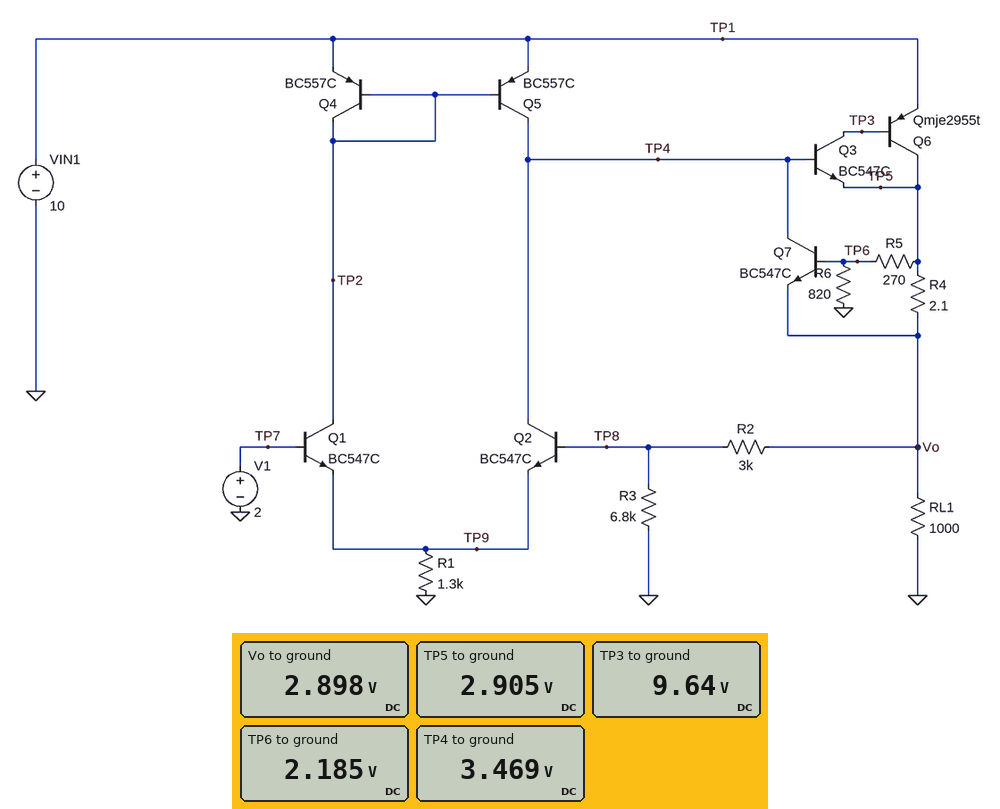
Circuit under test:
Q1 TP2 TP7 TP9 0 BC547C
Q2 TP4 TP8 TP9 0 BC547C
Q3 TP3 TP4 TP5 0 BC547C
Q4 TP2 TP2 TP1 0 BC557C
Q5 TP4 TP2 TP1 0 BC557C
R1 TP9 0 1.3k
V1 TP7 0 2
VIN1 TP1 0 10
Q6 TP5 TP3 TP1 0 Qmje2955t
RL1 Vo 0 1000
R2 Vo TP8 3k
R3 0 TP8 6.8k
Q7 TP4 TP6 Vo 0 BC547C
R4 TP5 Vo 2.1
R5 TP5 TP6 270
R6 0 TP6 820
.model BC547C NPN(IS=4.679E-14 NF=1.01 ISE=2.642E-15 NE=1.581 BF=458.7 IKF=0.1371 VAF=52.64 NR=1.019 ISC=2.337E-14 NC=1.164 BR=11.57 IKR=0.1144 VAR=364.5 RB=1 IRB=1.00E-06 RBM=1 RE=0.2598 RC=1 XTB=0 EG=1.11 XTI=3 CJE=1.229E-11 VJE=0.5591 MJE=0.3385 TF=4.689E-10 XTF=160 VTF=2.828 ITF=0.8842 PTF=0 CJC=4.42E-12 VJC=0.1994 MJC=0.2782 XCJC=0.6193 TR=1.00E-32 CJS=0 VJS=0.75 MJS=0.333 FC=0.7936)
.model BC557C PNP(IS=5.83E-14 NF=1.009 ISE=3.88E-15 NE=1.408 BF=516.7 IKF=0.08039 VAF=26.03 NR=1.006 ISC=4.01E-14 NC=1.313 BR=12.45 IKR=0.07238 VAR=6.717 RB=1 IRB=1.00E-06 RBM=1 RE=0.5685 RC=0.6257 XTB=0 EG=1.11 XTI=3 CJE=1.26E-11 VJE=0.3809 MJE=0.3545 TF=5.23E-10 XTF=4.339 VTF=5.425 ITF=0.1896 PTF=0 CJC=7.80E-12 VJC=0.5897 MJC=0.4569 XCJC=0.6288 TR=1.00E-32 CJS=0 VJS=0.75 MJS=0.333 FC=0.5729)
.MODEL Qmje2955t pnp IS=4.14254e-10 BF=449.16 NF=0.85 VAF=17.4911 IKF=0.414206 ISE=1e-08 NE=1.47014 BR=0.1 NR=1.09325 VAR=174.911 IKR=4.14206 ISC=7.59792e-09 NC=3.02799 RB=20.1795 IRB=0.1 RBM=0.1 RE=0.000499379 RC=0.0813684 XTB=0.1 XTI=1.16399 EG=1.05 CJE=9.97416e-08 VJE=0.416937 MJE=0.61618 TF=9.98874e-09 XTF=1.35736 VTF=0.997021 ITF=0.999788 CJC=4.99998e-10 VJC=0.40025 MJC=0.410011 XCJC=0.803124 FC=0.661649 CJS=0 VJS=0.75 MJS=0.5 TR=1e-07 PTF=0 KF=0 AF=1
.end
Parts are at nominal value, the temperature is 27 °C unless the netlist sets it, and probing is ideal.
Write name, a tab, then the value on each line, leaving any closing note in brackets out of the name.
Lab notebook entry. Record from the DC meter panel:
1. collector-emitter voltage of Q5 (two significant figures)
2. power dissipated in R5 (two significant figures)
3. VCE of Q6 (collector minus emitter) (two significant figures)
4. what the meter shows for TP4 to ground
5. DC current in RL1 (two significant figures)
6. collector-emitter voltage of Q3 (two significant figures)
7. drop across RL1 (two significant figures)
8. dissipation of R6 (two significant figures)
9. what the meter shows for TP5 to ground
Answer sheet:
collector-emitter voltage of Q5	-6.5 V
power dissipated in R5	1.9 mW
VCE of Q6 (collector minus emitter)	-7.1 V
what the meter shows for TP4 to ground	3.469 V
DC current in RL1	2.9 mA
collector-emitter voltage of Q3	6.7 V
drop across RL1	2.9 V
dissipation of R6	5.8 mW
what the meter shows for TP5 to ground	2.905 V
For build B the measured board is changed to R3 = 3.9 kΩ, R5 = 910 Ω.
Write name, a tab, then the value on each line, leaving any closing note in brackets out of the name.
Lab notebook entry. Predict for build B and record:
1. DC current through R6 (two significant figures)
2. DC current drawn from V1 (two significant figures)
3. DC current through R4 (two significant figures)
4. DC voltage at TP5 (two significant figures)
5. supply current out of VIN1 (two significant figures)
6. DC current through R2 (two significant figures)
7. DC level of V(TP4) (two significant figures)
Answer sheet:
DC current through R6	2.1 mA
DC current drawn from V1	940 nA
DC current through R4	4.1 mA
DC voltage at TP5	3.6 V
supply current out of VIN1	7.2 mA
DC current through R2	520 µA
DC level of V(TP4)	4.1 V
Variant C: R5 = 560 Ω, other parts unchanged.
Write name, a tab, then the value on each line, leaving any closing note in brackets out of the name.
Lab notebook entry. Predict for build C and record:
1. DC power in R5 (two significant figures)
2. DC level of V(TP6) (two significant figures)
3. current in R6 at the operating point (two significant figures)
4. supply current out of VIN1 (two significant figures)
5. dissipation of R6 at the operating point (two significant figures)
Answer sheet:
DC power in R5	2.5 mW
DC level of V(TP6)	1.7 V
current in R6 at the operating point	2.1 mA
supply current out of VIN1	6.4 mA
dissipation of R6 at the operating point	3.6 mW
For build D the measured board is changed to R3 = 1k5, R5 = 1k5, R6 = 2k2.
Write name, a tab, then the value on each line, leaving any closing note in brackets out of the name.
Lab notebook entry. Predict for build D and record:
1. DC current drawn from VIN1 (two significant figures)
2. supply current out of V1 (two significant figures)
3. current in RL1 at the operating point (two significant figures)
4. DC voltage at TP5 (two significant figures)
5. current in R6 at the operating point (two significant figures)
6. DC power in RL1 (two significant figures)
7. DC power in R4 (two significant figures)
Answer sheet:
DC current drawn from VIN1	10 mA
supply current out of V1	980 nA
current in RL1 at the operating point	6.0 mA
DC voltage at TP5	6.0 V
current in R6 at the operating point	1.6 mA
DC power in RL1	36 mW
DC power in R4	110 µW
